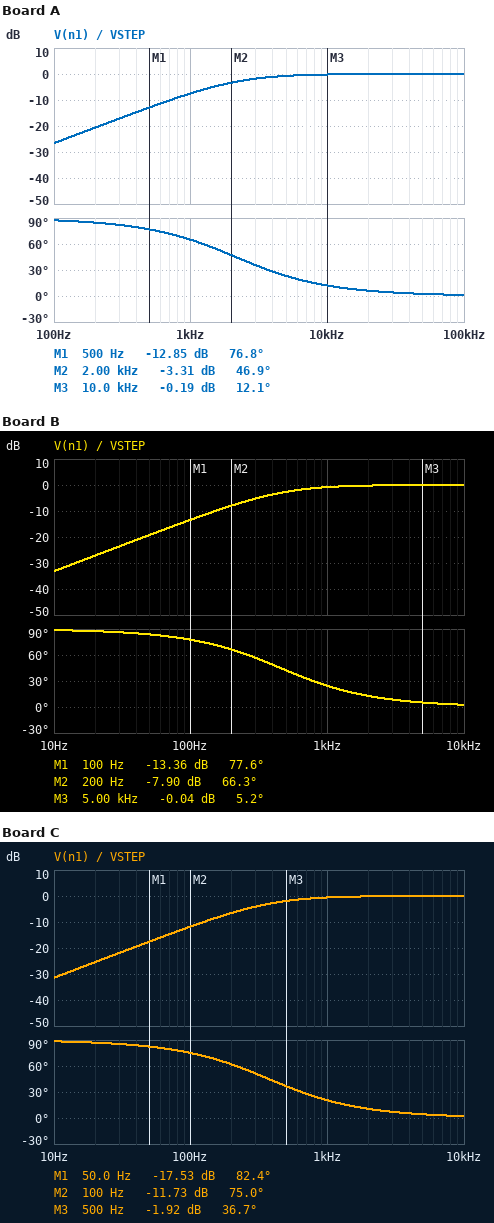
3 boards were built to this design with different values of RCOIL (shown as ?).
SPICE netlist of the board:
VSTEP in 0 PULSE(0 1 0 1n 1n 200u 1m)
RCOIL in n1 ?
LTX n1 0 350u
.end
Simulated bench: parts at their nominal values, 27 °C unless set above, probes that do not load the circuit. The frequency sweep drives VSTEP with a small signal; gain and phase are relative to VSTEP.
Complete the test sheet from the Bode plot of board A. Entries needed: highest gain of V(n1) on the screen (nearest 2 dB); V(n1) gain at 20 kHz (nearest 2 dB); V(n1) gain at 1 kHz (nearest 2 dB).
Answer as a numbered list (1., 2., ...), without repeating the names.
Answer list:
1. 0 dB
2. 0 dB
3. -8 dB
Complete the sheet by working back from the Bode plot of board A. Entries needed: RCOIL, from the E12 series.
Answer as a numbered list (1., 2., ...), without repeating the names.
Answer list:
1. 4.7 Ω
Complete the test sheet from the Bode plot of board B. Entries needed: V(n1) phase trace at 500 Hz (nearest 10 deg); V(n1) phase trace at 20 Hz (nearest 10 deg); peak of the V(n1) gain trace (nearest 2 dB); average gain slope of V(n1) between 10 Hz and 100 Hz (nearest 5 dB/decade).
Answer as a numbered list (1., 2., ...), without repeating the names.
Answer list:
1. 40 deg
2. 90 deg
3. 0 dB
4. 20 dB/decade
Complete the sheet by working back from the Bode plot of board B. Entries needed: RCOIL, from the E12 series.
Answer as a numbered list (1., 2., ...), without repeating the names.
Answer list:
1. 1 Ω
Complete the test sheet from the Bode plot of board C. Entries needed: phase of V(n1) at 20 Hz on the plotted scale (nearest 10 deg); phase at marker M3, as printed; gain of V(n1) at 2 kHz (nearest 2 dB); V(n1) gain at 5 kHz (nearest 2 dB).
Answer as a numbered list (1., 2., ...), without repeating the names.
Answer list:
1. 90 deg
2. 36.7 deg
3. 0 dB
4. 0 dB
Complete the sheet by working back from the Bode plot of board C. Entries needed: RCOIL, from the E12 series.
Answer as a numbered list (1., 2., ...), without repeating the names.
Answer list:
1. 0.82 Ω
